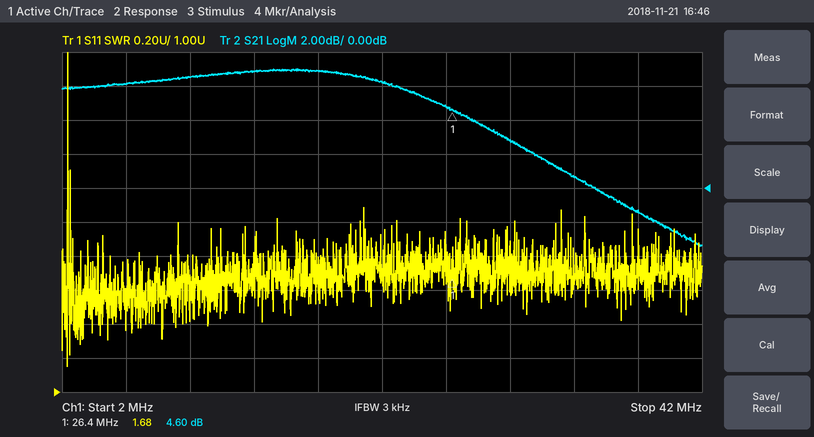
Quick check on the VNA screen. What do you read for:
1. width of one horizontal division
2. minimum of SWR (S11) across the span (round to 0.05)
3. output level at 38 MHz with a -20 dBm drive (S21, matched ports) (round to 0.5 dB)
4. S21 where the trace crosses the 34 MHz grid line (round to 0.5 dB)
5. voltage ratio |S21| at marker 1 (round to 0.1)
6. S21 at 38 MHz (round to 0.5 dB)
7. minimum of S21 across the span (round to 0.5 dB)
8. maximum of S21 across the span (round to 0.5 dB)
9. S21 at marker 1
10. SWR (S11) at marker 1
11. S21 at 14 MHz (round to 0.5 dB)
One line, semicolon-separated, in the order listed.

4 MHz; 1.15; -21.5 dBm; 0.5 dB; 1.7; -1.5 dB; -3.5 dB; 7.0 dB; 4.60 dB; 1.68; 7.0 dB
